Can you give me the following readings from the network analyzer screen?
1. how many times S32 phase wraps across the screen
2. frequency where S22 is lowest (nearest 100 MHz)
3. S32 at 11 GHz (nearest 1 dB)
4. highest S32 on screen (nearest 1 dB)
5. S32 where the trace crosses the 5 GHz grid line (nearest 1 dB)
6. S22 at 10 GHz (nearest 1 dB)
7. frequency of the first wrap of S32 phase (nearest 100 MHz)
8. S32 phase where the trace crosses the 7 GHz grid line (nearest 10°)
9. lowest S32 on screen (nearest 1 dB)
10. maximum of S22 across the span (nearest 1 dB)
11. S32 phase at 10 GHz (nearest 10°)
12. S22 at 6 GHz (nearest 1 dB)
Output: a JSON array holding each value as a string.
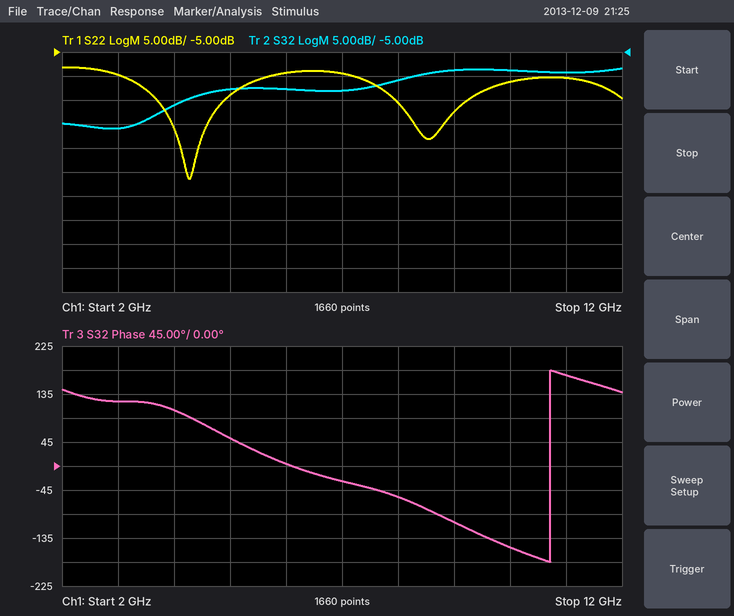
["1", "4.3 GHz", "-9 dB", "-8 dB", "-13 dB", "-11 dB", "10.7 GHz", "-30°", "-21 dB", "-8 dB", "-150°", "-9 dB"]
